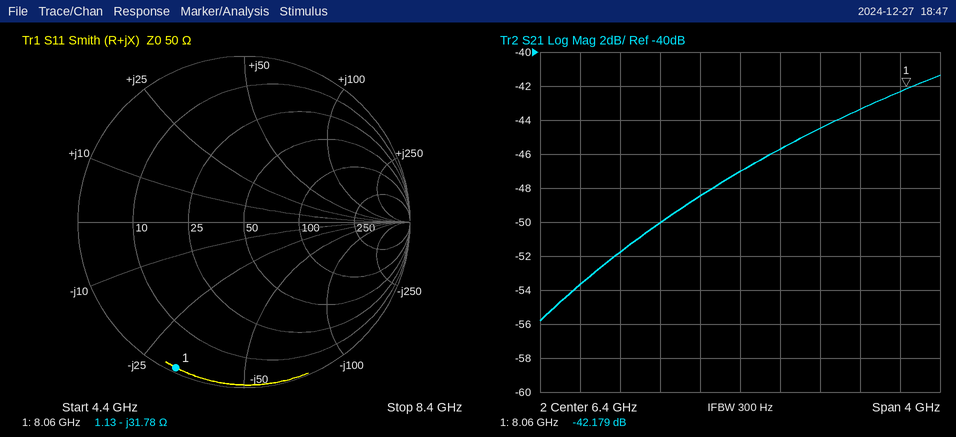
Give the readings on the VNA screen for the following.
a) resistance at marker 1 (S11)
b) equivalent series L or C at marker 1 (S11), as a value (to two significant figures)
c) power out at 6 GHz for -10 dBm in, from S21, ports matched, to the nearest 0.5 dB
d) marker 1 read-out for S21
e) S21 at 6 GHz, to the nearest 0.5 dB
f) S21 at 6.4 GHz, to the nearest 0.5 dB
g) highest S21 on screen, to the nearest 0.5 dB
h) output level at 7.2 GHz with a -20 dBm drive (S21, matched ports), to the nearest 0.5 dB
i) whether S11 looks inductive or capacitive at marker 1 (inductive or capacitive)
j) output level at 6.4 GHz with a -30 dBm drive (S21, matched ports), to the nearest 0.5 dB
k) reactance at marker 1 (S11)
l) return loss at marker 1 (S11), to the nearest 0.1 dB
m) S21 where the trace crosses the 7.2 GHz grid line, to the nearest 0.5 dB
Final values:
1.13 Ω
620 fF
-58.5 dBm
-42.179 dB
-48.5 dB
-47.0 dB
-41.5 dB
-64.5 dBm
capacitive
-77.0 dBm
-31.78 Ω
0.3 dB
-44.5 dB
